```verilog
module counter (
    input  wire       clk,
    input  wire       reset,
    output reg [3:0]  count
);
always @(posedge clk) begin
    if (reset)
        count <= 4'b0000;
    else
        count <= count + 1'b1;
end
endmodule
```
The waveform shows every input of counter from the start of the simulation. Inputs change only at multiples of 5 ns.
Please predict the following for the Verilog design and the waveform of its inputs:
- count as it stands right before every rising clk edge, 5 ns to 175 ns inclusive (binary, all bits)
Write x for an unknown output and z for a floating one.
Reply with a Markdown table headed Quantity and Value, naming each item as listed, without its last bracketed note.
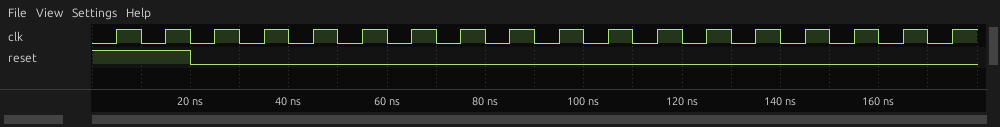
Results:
| Quantity | Value |
|---|---|
| count as it stands right before every rising clk edge, 5 ns to 175 ns inclusive | x, 0000, 0000, 0001, 0010, 0011, 0100, 0101, 0110, 0111, 1000, 1001, 1010, 1011, 1100, 1101, 1110, 1111 |
